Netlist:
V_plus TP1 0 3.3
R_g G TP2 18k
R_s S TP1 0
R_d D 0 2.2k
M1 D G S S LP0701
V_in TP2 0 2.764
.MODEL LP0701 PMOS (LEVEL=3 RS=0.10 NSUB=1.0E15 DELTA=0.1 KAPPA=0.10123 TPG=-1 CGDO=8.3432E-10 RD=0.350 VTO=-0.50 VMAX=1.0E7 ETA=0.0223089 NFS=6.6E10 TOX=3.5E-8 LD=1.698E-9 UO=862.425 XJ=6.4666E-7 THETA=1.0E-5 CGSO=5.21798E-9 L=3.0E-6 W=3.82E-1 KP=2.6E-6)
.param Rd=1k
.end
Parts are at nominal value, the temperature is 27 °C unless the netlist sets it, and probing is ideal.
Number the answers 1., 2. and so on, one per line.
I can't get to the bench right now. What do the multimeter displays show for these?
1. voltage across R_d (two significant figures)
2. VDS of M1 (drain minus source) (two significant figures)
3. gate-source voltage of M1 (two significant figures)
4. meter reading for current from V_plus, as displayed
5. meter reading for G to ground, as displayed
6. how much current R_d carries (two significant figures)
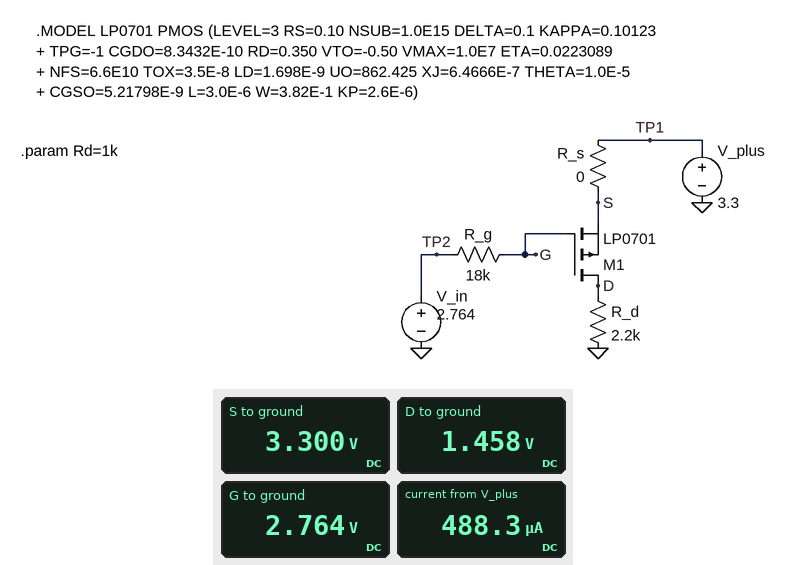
1. 1.5 V
2. -1.8 V
3. -540 mV
4. 488.3 µA
5. 2.764 V
6. 660 µA
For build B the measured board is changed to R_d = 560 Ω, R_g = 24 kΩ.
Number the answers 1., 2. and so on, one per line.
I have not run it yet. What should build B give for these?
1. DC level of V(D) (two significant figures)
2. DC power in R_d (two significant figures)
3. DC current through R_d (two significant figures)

1. 380 mV
2. 260 µW
3. 680 µA
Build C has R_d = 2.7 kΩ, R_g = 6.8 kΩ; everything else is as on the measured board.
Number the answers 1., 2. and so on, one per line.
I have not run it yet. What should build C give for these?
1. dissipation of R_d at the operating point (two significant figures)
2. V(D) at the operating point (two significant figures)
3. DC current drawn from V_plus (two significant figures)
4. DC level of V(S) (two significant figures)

1. 1.2 mW
2. 1.8 V
3. 980 µA
4. 3.3 V
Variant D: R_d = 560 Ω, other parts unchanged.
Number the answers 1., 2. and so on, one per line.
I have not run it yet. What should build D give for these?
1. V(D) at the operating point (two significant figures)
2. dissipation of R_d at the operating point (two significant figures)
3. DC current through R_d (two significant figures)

1. 380 mV
2. 260 µW
3. 680 µA
